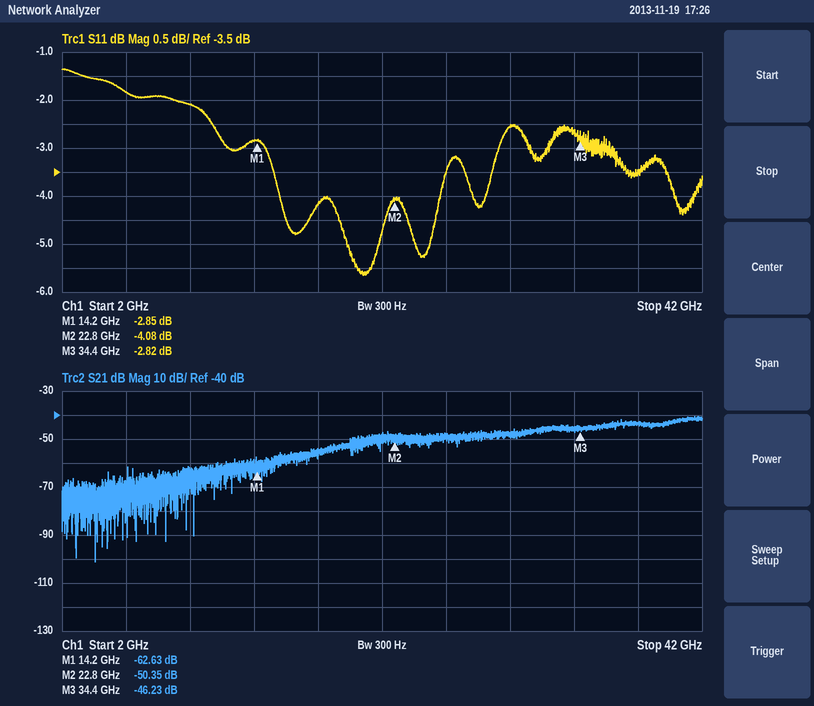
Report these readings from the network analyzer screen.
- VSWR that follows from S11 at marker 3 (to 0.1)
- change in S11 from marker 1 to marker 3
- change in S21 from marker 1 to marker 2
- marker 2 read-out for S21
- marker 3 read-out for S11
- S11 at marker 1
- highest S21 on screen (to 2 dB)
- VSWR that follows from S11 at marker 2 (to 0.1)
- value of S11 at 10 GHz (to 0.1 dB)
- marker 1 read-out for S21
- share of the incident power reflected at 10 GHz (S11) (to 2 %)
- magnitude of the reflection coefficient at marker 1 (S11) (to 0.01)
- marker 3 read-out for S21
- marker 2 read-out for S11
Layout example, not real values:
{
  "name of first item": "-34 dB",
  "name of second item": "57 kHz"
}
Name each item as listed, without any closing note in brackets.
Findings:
{
  "VSWR that follows from S11 at marker 3": "6.2",
  "change in S11 from marker 1 to marker 3": "0.03 dB",
  "change in S21 from marker 1 to marker 2": "12.28 dB",
  "marker 2 read-out for S21": "-50.35 dB",
  "marker 3 read-out for S11": "-2.82 dB",
  "S11 at marker 1": "-2.85 dB",
  "highest S21 on screen": "-40 dB",
  "VSWR that follows from S11 at marker 2": "4.3",
  "value of S11 at 10 GHz": "-2.1 dB",
  "marker 1 read-out for S21": "-62.63 dB",
  "share of the incident power reflected at 10 GHz (S11)": "62 %",
  "magnitude of the reflection coefficient at marker 1 (S11)": "0.72",
  "marker 3 read-out for S21": "-46.23 dB",
  "marker 2 read-out for S11": "-4.08 dB"
}
